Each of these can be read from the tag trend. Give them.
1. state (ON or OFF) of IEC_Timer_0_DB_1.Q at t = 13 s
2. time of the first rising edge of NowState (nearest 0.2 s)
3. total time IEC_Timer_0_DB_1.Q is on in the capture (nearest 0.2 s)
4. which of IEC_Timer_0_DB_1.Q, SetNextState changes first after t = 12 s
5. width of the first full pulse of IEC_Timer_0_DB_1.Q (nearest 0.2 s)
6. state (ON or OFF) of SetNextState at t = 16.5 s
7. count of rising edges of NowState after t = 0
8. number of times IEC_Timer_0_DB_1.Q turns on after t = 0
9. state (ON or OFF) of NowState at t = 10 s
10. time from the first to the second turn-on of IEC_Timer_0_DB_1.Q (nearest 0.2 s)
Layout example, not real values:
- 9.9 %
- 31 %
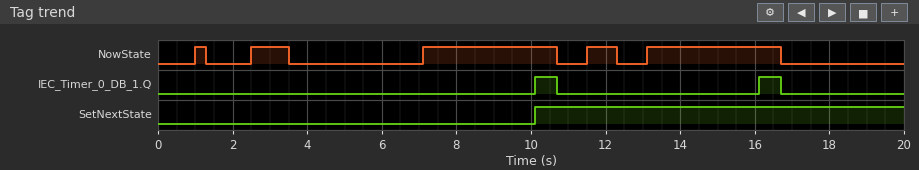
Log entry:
- OFF
- 1.0 s
- 1.2 s
- IEC_Timer_0_DB_1.Q
- 0.6 s
- ON
- 5
- 2
- ON
- 6.0 s
